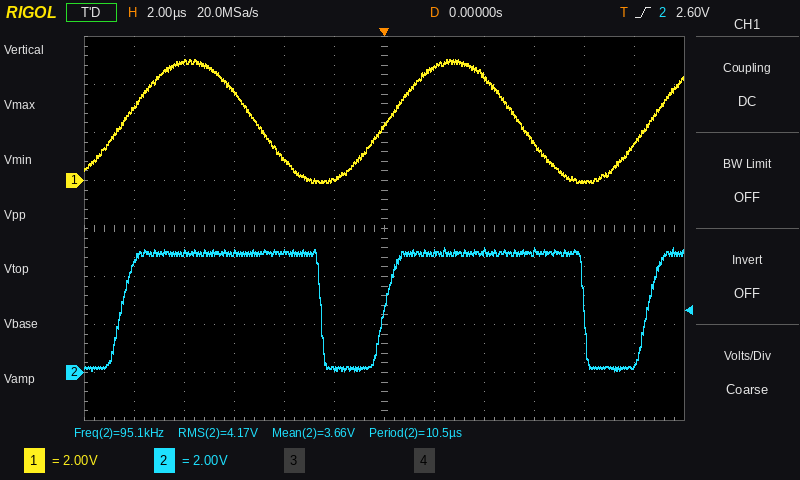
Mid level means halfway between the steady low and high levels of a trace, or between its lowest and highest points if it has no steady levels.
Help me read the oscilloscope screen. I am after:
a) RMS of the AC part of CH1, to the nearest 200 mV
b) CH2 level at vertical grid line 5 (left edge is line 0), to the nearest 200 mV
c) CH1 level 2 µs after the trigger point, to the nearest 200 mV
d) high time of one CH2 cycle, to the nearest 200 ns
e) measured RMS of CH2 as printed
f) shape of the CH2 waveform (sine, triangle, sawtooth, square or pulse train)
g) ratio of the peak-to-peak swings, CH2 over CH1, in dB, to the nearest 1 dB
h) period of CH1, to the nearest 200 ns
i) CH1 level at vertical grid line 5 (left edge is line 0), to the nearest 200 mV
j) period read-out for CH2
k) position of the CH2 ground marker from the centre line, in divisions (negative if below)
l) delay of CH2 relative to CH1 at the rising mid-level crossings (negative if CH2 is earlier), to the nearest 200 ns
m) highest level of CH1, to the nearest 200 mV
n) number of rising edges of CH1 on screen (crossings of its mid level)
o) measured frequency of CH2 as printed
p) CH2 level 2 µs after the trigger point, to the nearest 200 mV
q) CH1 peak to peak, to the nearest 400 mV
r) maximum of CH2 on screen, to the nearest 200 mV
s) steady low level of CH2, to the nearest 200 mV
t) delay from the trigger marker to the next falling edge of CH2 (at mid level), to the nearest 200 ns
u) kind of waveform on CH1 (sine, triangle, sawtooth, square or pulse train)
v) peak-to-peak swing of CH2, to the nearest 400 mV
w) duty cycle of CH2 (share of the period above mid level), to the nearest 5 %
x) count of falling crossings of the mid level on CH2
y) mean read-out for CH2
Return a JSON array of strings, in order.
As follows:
["1.8 V", "200 mV", "4.8 V", "8.0 µs", "4.17 V", "pulse train", "0 dB", "10.6 µs", "0.0 V", "10.5 µs", "-3.0 div", "-200 ns", "5.0 V", "3", "95.1 kHz", "5.0 V", "5.2 V", "5.2 V", "200 mV", "8.0 µs", "sine", "5.2 V", "75 %", "2", "3.66 V"]
